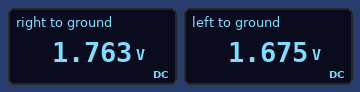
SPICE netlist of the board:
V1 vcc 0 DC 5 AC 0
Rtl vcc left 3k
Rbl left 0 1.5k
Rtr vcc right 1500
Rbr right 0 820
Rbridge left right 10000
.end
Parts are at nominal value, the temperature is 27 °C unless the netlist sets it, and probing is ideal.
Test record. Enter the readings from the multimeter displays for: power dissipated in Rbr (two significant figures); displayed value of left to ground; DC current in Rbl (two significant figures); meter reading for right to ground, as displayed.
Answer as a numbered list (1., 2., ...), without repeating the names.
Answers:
1. 3.8 mW
2. 1.675 V
3. 1.1 mA
4. 1.763 V
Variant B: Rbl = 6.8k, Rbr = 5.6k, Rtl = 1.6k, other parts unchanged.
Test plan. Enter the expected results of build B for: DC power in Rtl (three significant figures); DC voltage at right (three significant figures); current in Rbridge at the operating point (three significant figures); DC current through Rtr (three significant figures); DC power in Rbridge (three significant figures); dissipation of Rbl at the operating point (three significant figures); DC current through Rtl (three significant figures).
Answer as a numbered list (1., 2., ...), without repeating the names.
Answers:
1. 580 µW
2. 3.95 V
3. 8.33 µA
4. 698 µA
5. 694 nW
6. 2.40 mW
7. 602 µA
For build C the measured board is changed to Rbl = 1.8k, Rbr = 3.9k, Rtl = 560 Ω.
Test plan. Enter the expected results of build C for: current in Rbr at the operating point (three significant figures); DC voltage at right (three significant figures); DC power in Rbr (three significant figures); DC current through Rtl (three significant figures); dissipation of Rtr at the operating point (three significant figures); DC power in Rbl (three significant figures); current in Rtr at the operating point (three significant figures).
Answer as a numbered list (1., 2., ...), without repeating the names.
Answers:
1. 931 µA
2. 3.63 V
3. 3.38 mW
4. 2.13 mA
5. 1.25 mW
6. 8.05 mW
7. 913 µA
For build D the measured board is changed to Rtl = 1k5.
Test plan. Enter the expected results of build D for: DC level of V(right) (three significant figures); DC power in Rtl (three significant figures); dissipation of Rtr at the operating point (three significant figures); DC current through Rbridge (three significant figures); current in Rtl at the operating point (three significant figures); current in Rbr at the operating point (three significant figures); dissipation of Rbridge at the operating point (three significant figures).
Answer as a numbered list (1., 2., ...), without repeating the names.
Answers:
1. 1.80 V
2. 4.33 mW
3. 6.82 mW
4. 65.0 µA
5. 1.70 mA
6. 2.20 mA
7. 42.2 µW
